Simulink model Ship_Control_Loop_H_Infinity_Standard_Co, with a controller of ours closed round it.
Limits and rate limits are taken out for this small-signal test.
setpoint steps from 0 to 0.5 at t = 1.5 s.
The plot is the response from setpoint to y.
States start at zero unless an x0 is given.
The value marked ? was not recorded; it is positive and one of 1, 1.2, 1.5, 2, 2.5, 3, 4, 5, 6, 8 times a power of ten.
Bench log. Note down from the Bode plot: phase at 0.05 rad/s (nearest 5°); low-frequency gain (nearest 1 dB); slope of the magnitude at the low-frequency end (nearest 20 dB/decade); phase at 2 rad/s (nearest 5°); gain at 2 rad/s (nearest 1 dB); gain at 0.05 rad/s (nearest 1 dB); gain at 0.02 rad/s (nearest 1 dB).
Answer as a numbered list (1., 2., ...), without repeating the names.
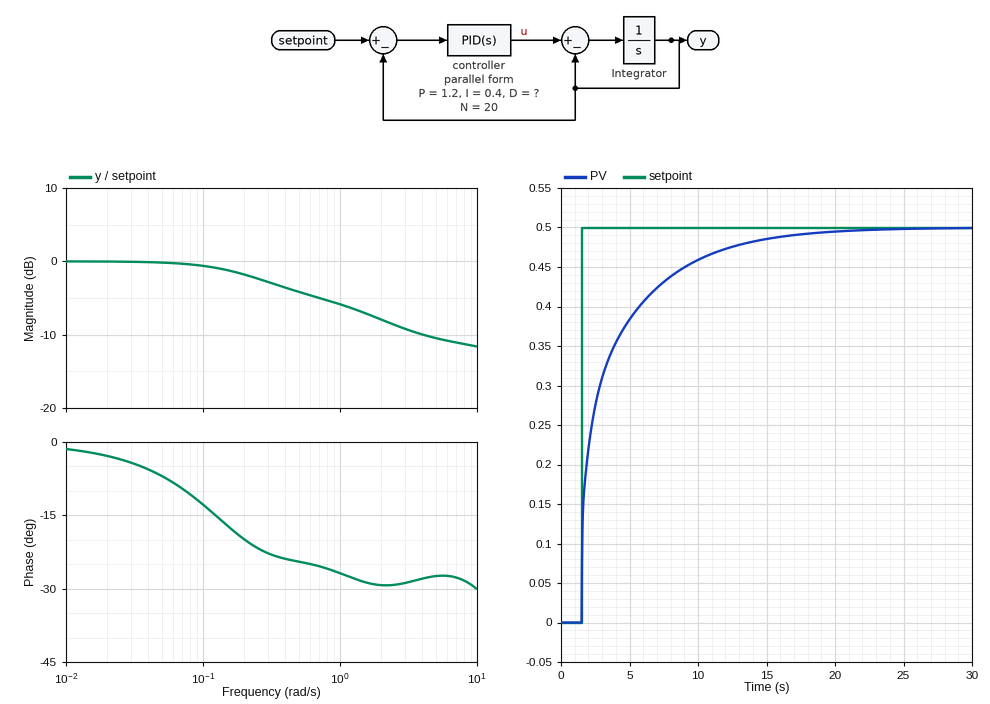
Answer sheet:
1. -5°
2. 0 dB
3. 0 dB/decade
4. -30°
5. -8 dB
6. 0 dB
7. 0 dB
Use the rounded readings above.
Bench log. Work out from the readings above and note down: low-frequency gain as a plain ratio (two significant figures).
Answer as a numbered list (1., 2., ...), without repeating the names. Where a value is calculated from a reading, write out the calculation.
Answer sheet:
1. 10^(0 / 20) = 1.0
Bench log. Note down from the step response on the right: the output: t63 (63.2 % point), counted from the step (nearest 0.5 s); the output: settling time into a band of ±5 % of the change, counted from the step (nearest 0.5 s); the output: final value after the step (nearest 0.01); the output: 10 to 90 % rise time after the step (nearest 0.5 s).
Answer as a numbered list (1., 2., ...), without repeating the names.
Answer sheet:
1. 1.5 s
2. 11.0 s
3. 0.50
4. 7.5 s
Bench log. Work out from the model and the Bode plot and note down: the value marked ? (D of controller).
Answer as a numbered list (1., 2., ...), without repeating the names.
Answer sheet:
1. 0.3
